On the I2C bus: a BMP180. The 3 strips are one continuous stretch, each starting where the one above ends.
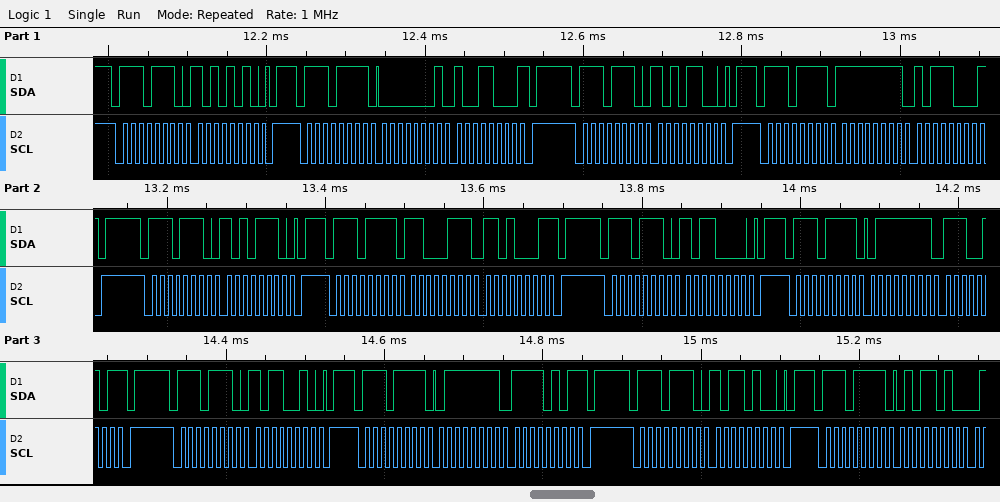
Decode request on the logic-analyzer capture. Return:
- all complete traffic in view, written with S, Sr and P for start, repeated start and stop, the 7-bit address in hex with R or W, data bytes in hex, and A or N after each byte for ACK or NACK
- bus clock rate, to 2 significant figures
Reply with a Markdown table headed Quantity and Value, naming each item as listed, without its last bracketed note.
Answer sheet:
| Quantity | Value |
|---|---|
| all complete traffic in view, written with S, Sr and P for start, repeated start and stop, the 7-bit address in hex with R or W, data bytes in hex, and A or N after each byte for ACK or NACK | S 77W A AA A P S 77R A 01 A 98 N P S 77W A AC A P S 77R A FF A B8 N P S 77W A AE A P S 77R A C7 A D1 N P S 77W A B0 A P S 77R A 7F A E5 N P S 77W A B2 A P S 77R A 7F A F5 N P S 77W A B4 A P S 77R A 5A A |
| bus clock rate, to 2 significant figures | 100 kHz |
